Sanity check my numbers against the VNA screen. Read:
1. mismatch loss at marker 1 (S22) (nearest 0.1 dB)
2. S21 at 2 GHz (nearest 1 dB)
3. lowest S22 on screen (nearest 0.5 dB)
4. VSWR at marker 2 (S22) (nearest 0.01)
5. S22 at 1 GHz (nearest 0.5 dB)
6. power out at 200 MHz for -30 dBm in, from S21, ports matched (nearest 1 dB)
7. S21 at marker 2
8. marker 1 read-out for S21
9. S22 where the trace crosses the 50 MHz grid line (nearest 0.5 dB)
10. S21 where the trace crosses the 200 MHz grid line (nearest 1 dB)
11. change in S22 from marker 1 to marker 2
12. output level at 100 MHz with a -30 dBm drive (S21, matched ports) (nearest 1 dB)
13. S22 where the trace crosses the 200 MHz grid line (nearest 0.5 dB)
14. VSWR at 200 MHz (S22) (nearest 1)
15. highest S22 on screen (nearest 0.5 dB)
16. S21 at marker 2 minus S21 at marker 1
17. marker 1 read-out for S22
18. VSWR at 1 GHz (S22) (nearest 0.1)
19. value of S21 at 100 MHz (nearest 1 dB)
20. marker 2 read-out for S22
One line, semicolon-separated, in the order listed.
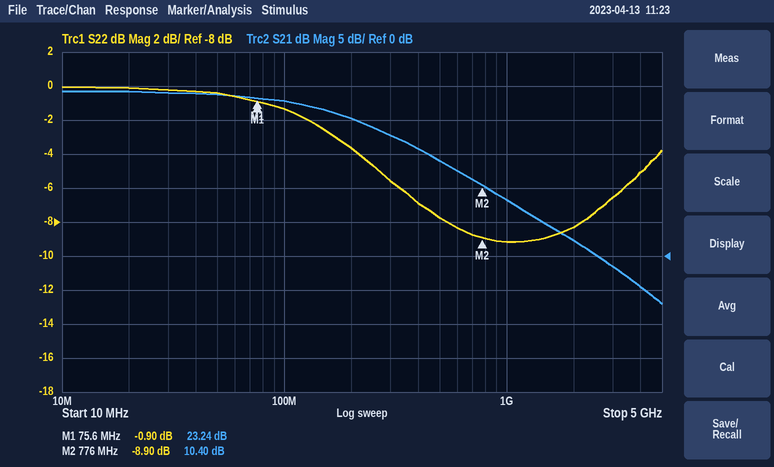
7.3 dB; 2 dB; -9.0 dB; 2.12; -9.0 dB; -10 dBm; 10.40 dB; 23.24 dB; -0.5 dB; 20 dB; -8.00 dB; -7 dBm; -3.5 dB; 5; 0.0 dB; -12.84 dB; -0.90 dB; 2.1; 23 dB; -8.90 dB
